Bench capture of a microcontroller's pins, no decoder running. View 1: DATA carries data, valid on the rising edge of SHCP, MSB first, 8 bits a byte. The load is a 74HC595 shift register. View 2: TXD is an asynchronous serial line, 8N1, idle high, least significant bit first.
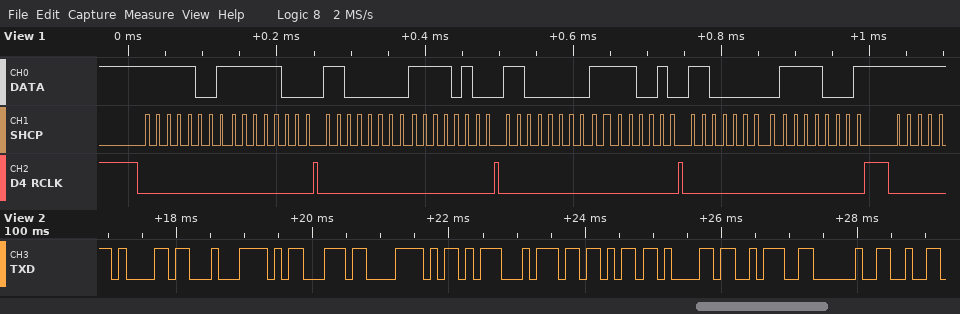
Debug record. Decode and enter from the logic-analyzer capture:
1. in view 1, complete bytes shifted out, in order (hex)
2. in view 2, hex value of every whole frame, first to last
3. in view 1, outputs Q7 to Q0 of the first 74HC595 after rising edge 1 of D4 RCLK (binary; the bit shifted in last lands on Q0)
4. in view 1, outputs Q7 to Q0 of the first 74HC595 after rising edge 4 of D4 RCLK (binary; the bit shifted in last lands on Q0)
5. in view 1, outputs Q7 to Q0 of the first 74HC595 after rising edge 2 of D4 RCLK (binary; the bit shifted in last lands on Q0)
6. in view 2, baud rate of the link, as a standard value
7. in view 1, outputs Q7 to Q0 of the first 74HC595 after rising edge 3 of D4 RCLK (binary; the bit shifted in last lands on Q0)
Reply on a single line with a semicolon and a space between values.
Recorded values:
F9 F8 C0 F4 C0 F2 C0 F1; 61 C4 8D C3 AD 74 6B 61 3A 20; 11111000; 11110001; 11110100; 9600 baud; 11110010
